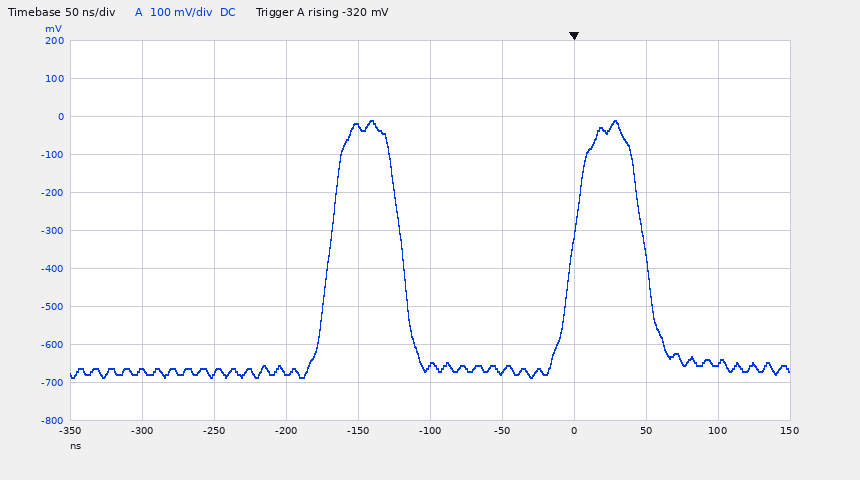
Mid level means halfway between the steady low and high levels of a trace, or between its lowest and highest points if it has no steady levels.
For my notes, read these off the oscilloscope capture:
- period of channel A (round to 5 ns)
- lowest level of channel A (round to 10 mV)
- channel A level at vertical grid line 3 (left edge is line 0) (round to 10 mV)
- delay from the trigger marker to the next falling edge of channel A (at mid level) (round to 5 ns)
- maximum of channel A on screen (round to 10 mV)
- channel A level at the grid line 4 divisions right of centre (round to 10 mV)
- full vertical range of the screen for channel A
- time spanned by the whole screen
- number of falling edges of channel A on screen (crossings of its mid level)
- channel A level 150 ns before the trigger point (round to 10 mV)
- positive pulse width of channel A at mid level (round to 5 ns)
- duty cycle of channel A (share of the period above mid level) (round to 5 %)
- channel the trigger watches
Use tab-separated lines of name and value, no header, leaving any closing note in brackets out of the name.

period of channel A	170 ns
lowest level of channel A	-690 mV
channel A level at vertical grid line 3 (left edge is line 0)	-670 mV
delay from the trigger marker to the next falling edge of channel A (at mid level)	50 ns
maximum of channel A on screen	-10 mV
channel A level at the grid line 4 divisions right of centre	-650 mV
full vertical range of the screen for channel A	1 V
time spanned by the whole screen	500 ns
number of falling edges of channel A on screen	2
channel A level 150 ns before the trigger point	-30 mV
positive pulse width of channel A at mid level	50 ns
duty cycle of channel A (share of the period above mid level)	30 %
channel the trigger watches	channel A
